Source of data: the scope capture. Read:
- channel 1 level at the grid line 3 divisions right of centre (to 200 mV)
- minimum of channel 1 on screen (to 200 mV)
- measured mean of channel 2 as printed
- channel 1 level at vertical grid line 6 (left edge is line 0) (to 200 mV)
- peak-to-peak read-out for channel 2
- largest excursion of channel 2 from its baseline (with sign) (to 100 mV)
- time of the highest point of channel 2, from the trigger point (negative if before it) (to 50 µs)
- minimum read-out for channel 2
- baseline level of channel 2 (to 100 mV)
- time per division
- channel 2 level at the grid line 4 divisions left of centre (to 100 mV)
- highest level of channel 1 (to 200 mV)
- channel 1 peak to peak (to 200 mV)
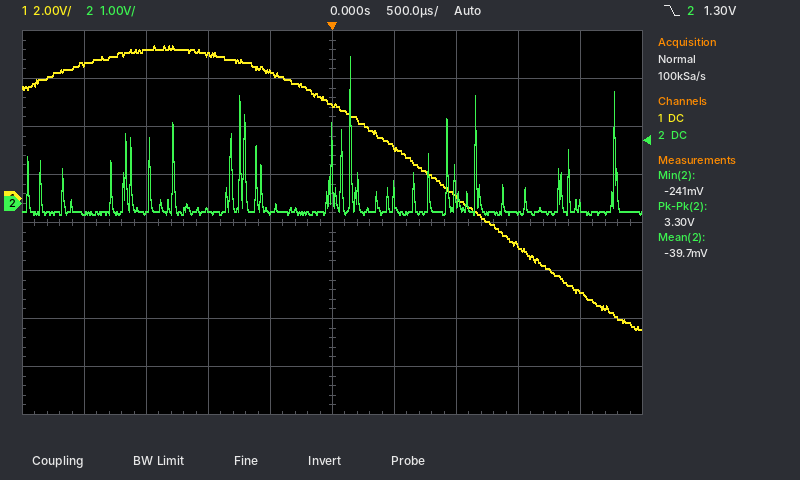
-2.0 V
-5.4 V
-39.7 mV
2.2 V
3.30 V
+3.2 V
+150 µs
-241 mV
-200 mV
500 µs
-200 mV
6.4 V
11.8 V
